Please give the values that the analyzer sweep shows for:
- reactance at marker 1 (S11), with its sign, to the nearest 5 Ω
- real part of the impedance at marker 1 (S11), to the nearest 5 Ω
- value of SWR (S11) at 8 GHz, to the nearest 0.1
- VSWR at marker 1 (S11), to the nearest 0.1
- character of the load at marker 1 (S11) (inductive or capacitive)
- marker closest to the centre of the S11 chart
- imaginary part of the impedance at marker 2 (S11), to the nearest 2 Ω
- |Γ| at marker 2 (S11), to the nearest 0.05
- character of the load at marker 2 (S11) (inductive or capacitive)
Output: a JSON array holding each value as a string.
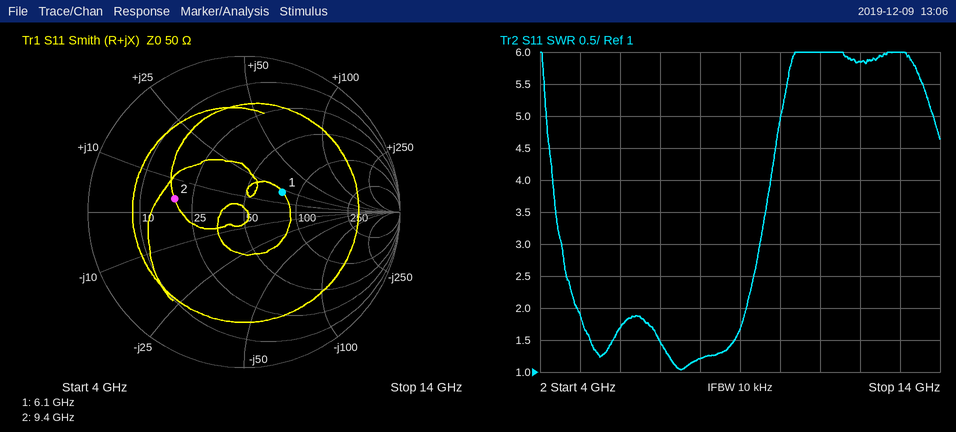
["+20 Ω", "80 Ω", "1.2", "1.8", "inductive", "marker 1", "+4 Ω", "0.45", "inductive"]
